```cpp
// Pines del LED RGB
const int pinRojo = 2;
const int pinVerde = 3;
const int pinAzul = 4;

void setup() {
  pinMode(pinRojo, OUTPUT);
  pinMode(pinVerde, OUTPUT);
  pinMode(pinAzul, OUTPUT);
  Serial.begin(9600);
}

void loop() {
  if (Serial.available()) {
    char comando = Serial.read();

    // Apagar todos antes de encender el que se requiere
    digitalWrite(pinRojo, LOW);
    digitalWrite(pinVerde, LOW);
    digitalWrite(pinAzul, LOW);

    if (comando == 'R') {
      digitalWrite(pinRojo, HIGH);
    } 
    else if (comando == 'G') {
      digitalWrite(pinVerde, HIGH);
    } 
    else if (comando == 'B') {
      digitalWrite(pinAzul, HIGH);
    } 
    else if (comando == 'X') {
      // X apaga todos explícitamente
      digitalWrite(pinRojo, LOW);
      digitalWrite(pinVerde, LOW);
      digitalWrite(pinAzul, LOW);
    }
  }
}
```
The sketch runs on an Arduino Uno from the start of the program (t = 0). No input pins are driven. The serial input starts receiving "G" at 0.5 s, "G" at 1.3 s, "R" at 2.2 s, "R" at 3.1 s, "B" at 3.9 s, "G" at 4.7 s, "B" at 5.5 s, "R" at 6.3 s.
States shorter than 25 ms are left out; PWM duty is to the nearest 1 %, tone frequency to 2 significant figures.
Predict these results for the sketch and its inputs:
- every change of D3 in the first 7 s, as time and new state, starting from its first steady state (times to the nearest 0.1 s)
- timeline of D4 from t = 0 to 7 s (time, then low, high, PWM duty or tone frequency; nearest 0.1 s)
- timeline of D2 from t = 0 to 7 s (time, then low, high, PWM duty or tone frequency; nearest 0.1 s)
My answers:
0 s low; 0.5 s high; 2.2 s low; 4.7 s high; 5.5 s low
0 s low; 3.9 s high; 4.7 s low; 5.5 s high; 6.3 s low
0 s low; 2.2 s high; 3.9 s low; 6.3 s high
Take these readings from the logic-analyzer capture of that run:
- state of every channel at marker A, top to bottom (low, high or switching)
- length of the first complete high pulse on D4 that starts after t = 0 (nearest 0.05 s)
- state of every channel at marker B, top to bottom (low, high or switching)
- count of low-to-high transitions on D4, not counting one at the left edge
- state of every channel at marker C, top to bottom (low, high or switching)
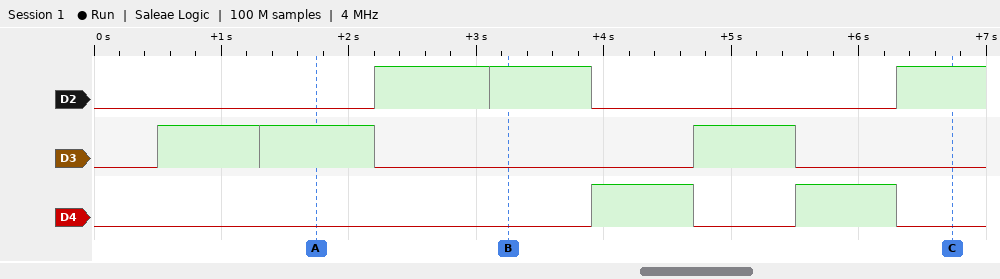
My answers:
D2 low, D3 high, D4 low
0.80 s
D2 high, D3 low, D4 low
2
D2 high, D3 low, D4 low
